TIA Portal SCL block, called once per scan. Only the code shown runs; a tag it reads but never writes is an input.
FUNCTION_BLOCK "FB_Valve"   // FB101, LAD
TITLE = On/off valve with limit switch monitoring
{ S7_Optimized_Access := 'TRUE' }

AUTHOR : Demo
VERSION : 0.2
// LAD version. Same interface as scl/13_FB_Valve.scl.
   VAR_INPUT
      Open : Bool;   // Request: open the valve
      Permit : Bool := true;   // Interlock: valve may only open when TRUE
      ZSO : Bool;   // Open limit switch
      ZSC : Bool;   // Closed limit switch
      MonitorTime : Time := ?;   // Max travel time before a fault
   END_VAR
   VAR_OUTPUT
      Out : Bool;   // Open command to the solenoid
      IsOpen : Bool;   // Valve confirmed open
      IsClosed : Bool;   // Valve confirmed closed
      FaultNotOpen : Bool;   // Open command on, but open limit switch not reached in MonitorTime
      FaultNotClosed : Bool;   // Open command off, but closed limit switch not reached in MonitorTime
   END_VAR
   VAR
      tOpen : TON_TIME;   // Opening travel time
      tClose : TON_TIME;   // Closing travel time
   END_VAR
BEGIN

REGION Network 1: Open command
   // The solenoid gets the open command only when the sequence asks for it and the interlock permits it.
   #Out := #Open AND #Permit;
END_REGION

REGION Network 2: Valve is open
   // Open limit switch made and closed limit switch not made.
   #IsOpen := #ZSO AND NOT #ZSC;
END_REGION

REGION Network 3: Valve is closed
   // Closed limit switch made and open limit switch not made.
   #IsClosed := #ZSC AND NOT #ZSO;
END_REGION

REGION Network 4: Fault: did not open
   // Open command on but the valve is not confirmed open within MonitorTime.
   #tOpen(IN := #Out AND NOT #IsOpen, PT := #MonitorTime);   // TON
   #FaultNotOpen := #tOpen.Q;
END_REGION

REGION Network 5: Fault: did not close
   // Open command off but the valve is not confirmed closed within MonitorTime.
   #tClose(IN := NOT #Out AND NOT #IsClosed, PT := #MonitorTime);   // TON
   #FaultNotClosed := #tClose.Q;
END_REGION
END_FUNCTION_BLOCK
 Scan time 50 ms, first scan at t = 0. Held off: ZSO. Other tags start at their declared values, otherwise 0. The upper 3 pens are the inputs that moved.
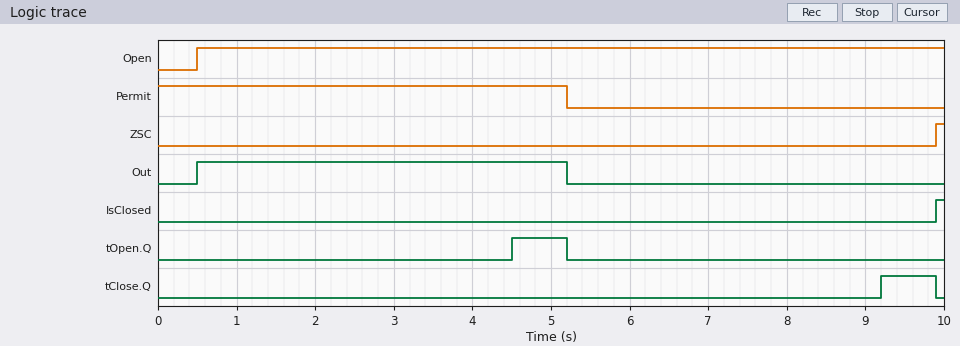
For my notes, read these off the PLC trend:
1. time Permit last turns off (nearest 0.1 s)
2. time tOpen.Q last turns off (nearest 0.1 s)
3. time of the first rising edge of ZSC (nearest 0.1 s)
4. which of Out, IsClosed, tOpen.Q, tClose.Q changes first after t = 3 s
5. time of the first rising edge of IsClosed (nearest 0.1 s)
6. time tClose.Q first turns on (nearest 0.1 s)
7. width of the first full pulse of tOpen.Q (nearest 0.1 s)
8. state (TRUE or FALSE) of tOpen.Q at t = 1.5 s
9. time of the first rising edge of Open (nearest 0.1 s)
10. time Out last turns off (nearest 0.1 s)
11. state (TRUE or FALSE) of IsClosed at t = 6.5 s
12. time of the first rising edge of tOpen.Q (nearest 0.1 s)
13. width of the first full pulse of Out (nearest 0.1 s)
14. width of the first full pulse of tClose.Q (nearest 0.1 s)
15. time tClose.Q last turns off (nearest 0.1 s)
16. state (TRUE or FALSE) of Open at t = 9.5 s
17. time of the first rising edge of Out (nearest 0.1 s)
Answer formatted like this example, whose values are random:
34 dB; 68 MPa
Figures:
5.2 s; 5.2 s; 9.9 s; tOpen.Q; 9.9 s; 9.2 s; 0.7 s; FALSE; 0.5 s; 5.2 s; FALSE; 4.5 s; 4.7 s; 0.7 s; 9.9 s; TRUE; 0.5 s
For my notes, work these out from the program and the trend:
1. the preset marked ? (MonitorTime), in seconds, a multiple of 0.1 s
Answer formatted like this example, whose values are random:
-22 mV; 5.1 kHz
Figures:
4.0 s
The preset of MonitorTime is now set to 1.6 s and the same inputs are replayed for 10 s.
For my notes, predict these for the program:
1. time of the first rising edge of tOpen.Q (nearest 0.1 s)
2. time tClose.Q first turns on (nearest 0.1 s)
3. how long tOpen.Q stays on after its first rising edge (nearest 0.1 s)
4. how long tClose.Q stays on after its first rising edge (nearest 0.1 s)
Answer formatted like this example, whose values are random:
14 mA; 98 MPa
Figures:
2.1 s; 6.8 s; 3.1 s; 3.1 s
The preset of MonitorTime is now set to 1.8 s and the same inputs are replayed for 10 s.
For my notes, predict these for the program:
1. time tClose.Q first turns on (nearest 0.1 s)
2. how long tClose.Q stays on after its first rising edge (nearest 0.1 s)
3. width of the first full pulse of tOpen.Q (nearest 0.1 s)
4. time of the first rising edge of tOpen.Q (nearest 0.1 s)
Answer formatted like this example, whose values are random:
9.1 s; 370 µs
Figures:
7.0 s; 2.9 s; 2.9 s; 2.3 s
